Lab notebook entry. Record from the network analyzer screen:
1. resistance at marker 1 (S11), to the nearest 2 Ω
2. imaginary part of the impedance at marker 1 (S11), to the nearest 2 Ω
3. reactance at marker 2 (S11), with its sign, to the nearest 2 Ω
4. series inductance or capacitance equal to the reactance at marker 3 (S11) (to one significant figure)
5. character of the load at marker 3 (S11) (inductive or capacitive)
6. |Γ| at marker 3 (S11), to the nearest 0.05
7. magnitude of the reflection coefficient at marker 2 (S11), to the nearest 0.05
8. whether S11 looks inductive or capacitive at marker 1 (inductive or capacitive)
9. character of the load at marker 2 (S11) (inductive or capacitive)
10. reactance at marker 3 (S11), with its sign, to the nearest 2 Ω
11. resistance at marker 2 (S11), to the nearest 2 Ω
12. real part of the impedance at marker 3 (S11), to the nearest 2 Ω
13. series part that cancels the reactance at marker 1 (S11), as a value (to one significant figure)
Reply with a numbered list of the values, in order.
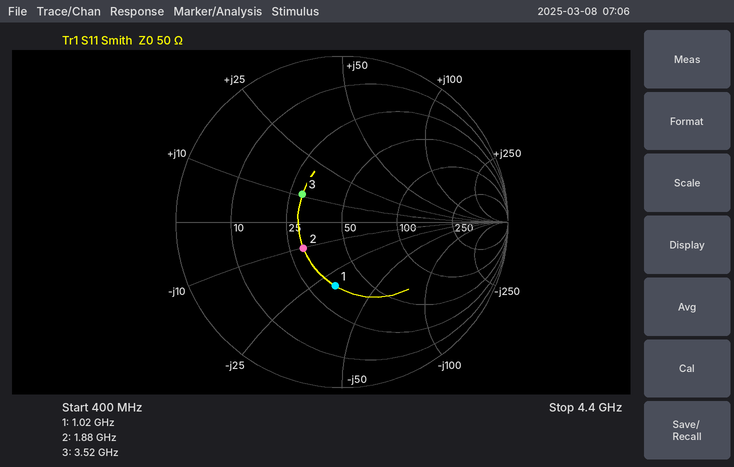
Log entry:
1. 34 Ω
2. -32 Ω
3. -10 Ω
4. 500 pH
5. inductive
6. 0.30
7. 0.30
8. capacitive
9. capacitive
10. +10 Ω
11. 30 Ω
12. 30 Ω
13. 5 nH
